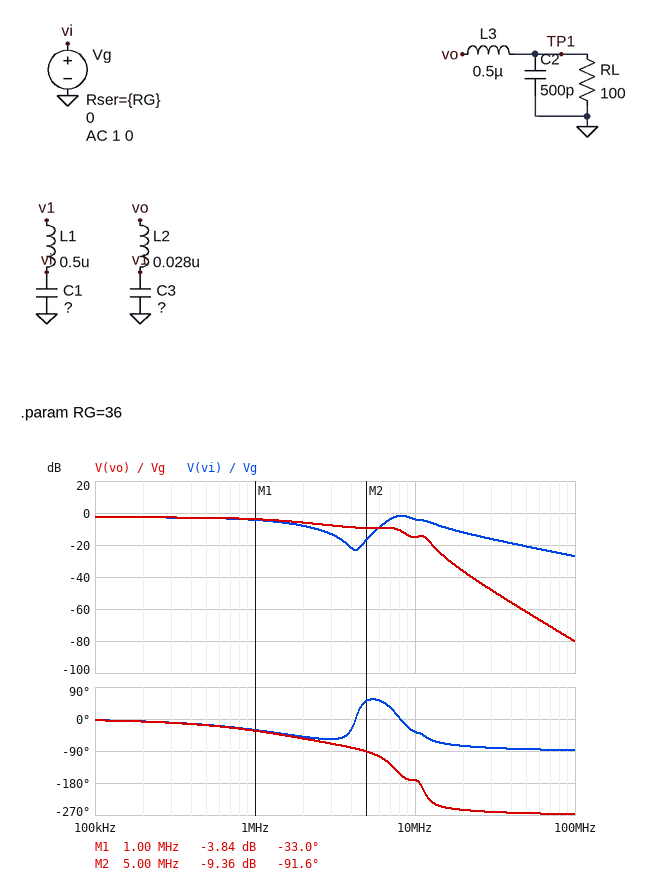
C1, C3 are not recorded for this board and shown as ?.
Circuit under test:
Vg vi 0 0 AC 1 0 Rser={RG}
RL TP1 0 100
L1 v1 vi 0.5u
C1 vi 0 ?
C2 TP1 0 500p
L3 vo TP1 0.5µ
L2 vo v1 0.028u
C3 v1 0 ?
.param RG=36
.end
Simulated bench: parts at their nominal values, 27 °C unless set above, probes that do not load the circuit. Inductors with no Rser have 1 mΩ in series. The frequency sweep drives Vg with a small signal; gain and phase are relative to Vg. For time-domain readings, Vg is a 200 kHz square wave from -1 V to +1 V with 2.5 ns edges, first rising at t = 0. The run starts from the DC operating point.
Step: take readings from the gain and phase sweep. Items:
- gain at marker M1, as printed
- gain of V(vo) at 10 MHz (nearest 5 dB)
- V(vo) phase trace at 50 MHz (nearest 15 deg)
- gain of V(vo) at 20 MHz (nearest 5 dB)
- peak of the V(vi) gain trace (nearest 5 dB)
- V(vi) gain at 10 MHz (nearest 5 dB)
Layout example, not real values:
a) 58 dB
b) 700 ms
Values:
a) -3.84 dB
b) -15 dB
c) -270 deg
d) -35 dB
e) 0 dB
f) -5 dB
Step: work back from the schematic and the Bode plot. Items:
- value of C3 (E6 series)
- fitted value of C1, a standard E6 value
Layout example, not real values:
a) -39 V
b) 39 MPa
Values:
a) 2.2 nF
b) 1 nF
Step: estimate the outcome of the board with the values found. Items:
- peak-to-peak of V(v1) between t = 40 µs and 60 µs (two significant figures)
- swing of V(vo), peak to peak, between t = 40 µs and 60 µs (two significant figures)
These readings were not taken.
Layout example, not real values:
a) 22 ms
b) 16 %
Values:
a) 1.5 V
b) 1.5 V
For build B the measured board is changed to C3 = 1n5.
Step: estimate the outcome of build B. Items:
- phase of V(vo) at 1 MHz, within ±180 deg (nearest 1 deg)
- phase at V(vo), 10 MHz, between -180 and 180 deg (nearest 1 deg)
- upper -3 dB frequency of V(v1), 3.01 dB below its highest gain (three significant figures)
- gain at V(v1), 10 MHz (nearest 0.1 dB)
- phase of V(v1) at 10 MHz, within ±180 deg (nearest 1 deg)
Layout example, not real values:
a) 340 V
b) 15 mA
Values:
a) -28 deg
b) -149 deg
c) 2.35 MHz
d) -13.9 dB
e) -140 deg
